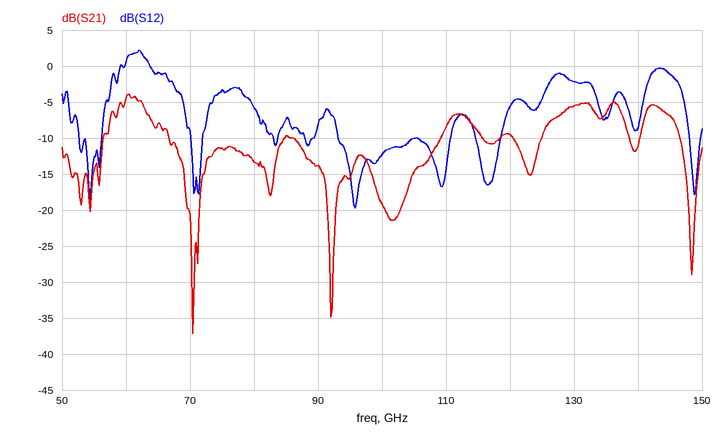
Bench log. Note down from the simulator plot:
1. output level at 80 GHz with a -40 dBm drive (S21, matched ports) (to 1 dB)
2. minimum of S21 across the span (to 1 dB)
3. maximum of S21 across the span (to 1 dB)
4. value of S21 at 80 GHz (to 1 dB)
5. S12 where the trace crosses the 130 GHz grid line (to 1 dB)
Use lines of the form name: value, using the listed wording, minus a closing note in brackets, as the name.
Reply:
output level at 80 GHz with a -40 dBm drive (S21, matched ports): -53 dBm
minimum of S21 across the span: -37 dB
maximum of S21 across the span: -4 dB
value of S21 at 80 GHz: -13 dB
S12 where the trace crosses the 130 GHz grid line: -2 dB
